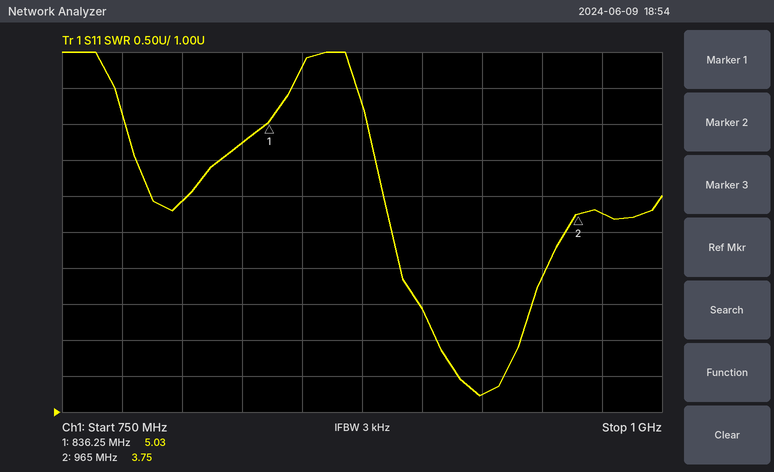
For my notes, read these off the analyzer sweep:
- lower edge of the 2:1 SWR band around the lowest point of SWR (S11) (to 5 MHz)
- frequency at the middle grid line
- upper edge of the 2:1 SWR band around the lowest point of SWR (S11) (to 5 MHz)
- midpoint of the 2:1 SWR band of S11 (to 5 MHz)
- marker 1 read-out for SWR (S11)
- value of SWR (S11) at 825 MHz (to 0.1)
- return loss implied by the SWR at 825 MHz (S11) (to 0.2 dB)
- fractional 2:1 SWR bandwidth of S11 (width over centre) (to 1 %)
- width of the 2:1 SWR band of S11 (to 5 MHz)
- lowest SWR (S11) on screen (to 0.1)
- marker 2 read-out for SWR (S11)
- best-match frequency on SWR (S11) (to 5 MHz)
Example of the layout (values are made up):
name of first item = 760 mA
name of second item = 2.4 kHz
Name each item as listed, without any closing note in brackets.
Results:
lower edge of the 2:1 SWR band around the lowest point of SWR (S11) = 905 MHz
frequency at the middle grid line = 875 MHz
upper edge of the 2:1 SWR band around the lowest point of SWR (S11) = 940 MHz
midpoint of the 2:1 SWR band of S11 = 925 MHz
marker 1 read-out for SWR = 5.03
value of SWR (S11) at 825 MHz = 4.7
return loss implied by the SWR at 825 MHz (S11) = 3.8 dB
fractional 2:1 SWR bandwidth of S11 (width over centre) = 4 %
width of the 2:1 SWR band of S11 = 35 MHz
lowest SWR (S11) on screen = 1.2
marker 2 read-out for SWR = 3.75
best-match frequency on SWR (S11) = 925 MHz
